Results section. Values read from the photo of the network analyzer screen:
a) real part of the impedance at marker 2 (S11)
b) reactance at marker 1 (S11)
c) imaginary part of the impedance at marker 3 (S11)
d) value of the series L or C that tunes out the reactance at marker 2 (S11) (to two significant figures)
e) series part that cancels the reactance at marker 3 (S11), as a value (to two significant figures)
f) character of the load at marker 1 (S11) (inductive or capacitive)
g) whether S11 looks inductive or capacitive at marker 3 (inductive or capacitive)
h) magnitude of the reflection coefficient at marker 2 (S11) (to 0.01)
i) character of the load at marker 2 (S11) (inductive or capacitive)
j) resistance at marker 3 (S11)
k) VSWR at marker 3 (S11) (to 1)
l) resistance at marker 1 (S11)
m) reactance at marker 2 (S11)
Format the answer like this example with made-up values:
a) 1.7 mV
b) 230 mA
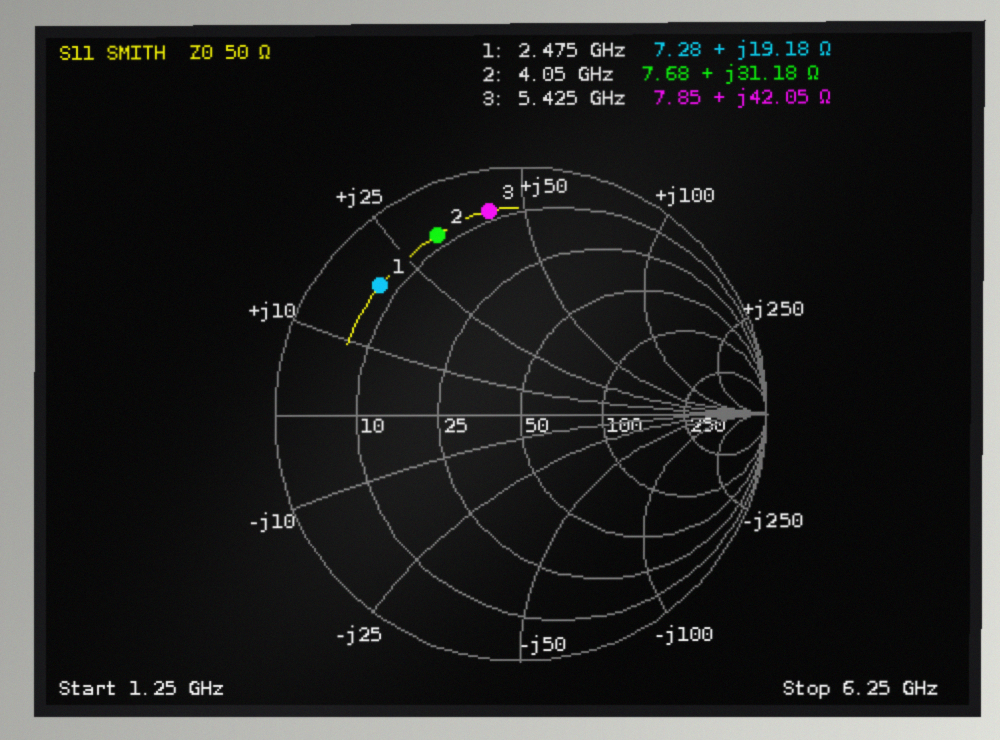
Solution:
a) 7.68 Ω
b) +19.18 Ω
c) +42.05 Ω
d) 1.3 pF
e) 700 fF
f) inductive
g) inductive
h) 0.80
i) inductive
j) 7.85 Ω
k) 11
l) 7.28 Ω
m) +31.18 Ω
